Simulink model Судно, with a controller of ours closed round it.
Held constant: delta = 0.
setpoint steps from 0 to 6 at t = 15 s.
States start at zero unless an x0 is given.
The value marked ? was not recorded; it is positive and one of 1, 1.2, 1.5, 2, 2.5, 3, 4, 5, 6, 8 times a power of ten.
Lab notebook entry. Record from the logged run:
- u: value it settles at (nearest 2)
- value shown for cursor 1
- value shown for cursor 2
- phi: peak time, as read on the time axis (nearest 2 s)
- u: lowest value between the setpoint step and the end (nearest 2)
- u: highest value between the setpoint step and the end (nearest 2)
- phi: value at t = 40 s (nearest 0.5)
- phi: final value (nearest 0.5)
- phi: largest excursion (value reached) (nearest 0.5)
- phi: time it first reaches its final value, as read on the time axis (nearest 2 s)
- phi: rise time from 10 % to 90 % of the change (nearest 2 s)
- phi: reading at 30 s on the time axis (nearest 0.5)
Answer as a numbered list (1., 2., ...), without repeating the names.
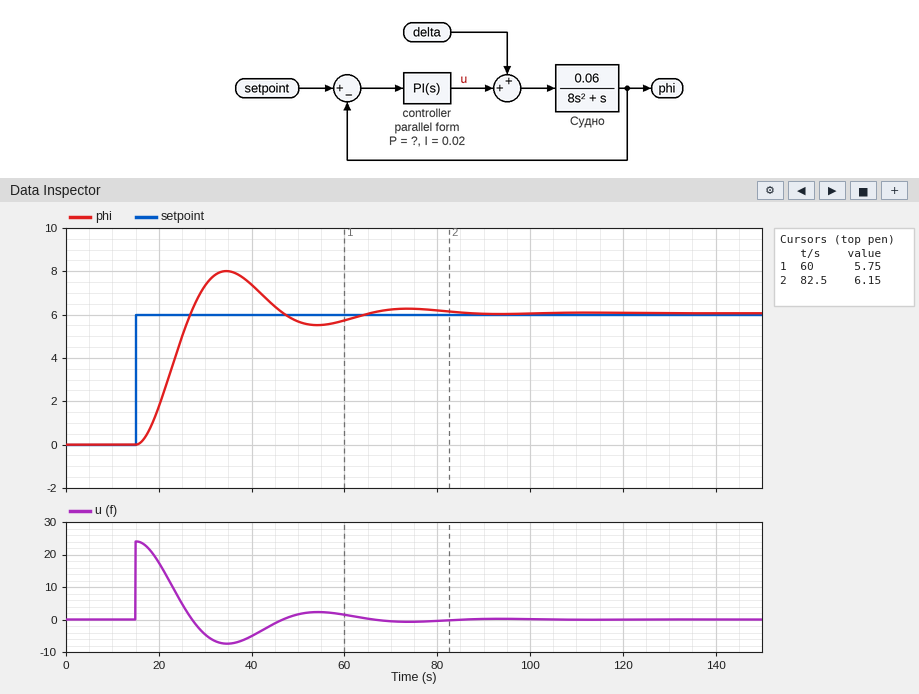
1. 0
2. 5.75
3. 6.15
4. 34 s
5. -8
6. 24
7. 7.5
8. 6.0
9. 8.0
10. 26 s
11. 8 s
12. 7.5
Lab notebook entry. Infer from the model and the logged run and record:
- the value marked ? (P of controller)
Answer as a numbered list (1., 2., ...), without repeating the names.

1. 4
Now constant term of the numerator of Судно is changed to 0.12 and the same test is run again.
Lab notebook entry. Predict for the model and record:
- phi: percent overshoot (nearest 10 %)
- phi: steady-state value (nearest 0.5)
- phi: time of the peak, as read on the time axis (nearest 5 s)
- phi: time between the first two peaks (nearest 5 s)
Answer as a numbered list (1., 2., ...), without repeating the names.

1. 50 %
2. 6.0
3. 30 s
4. 25 s
